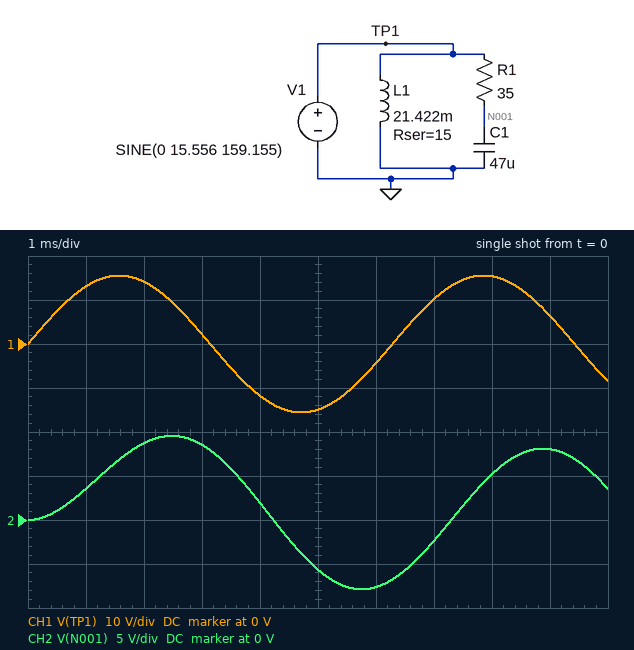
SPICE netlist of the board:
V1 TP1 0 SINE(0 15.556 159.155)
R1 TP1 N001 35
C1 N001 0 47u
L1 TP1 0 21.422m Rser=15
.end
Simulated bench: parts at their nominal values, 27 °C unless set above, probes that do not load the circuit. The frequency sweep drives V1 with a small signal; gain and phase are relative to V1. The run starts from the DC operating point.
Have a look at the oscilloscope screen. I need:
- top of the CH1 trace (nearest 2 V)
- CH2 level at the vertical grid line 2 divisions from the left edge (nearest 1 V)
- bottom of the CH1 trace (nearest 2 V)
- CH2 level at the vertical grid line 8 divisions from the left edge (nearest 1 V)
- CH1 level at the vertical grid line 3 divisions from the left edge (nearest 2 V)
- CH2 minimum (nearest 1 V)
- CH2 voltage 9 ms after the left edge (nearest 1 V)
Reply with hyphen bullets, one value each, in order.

- 16 V
- 9 V
- -16 V
- 5 V
- 2 V
- -8 V
- 8 V
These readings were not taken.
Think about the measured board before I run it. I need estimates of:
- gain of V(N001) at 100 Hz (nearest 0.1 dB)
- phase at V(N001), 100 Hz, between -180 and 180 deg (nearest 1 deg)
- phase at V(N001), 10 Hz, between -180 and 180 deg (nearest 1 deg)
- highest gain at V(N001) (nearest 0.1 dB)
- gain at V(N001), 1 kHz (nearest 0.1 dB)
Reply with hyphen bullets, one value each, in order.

- -3.2 dB
- -46 deg
- -6 deg
- 0 dB
- -20.3 dB
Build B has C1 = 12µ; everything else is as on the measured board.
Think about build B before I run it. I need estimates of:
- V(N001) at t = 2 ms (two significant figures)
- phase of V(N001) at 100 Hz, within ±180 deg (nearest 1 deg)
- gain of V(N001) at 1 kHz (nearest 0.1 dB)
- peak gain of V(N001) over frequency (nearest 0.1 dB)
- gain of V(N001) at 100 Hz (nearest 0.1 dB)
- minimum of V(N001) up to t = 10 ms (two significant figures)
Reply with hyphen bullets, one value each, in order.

- 14 V
- -15 deg
- -9.0 dB
- 0 dB
- -0.3 dB
- -14 V
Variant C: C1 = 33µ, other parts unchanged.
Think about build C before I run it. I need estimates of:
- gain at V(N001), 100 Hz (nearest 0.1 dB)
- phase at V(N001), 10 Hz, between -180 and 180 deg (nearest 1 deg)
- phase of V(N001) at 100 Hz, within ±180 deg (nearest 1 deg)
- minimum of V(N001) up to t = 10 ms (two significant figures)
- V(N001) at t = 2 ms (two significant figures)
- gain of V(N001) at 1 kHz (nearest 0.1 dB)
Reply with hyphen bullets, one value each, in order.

- -1.8 dB
- -4 deg
- -36 deg
- -10 V
- 11 V
- -17.3 dB
